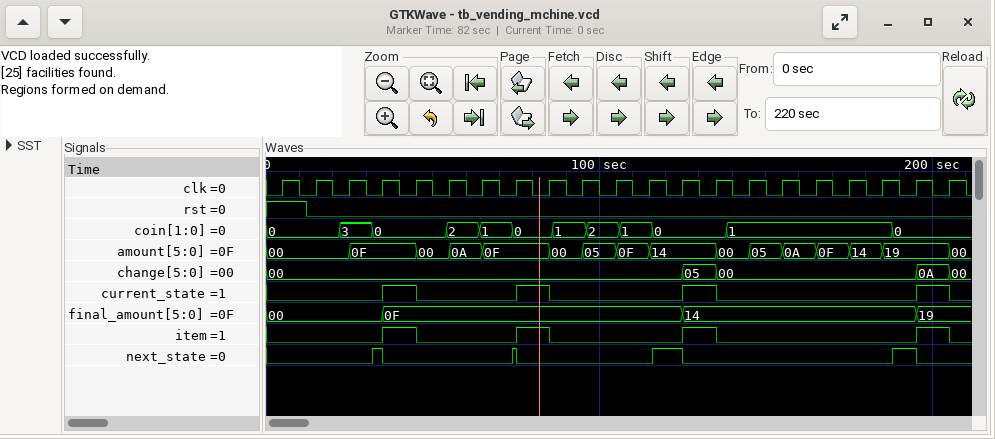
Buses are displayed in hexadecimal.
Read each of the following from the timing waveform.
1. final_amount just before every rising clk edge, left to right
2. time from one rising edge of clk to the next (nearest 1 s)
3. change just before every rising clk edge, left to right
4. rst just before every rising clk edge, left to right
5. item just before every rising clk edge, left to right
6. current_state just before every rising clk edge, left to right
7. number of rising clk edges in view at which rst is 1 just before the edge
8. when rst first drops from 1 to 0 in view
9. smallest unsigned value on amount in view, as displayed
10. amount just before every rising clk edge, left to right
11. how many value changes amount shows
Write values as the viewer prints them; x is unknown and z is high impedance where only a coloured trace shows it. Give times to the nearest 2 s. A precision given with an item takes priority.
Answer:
00, 00, 00, 00, 0F, 0F, 0F, 0F, 0F, 0F, 0F, 0F, 0F, 14, 14, 14, 14, 14, 14, 14, 19
10 s
00, 00, 00, 00, 00, 00, 00, 00, 00, 00, 00, 00, 00, 05, 00, 00, 00, 00, 00, 00, 0A
1 0 0 0 0 0 0 0 0 0 0 0 0 0 0 0 0 0 0 0 0
0 0 0 0 1 0 0 0 1 0 0 0 0 1 0 0 0 0 0 0 1
0 0 0 0 1 0 0 0 1 0 0 0 0 1 0 0 0 0 0 0 1
1
12 s
00
00, 00, 00, 0F, 0F, 00, 0A, 0F, 0F, 00, 05, 0F, 14, 14, 00, 05, 0A, 0F, 14, 19, 19
15
